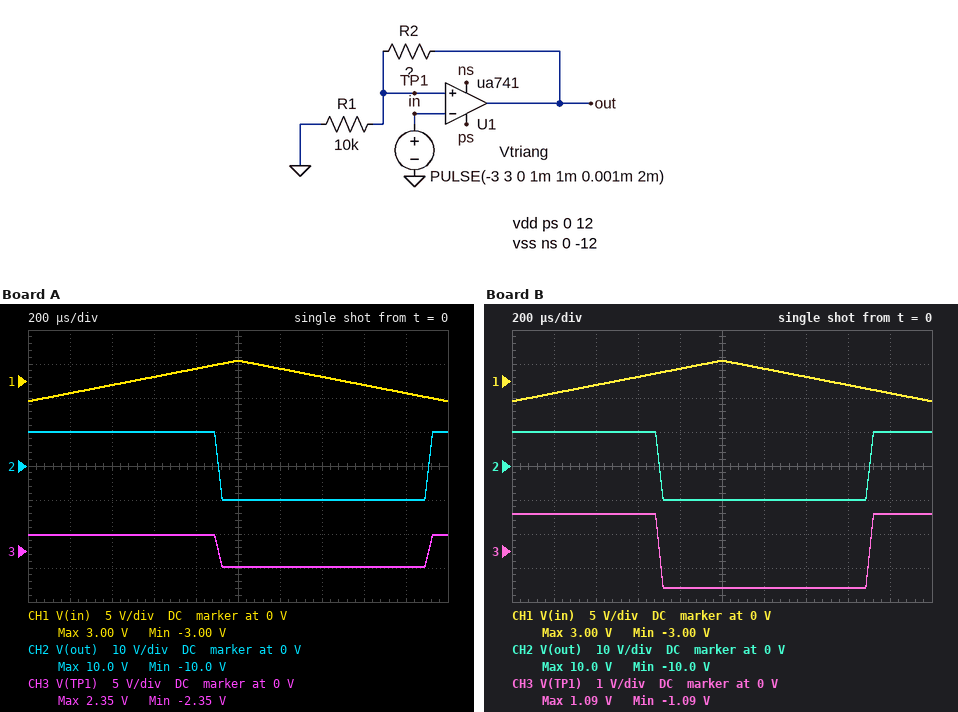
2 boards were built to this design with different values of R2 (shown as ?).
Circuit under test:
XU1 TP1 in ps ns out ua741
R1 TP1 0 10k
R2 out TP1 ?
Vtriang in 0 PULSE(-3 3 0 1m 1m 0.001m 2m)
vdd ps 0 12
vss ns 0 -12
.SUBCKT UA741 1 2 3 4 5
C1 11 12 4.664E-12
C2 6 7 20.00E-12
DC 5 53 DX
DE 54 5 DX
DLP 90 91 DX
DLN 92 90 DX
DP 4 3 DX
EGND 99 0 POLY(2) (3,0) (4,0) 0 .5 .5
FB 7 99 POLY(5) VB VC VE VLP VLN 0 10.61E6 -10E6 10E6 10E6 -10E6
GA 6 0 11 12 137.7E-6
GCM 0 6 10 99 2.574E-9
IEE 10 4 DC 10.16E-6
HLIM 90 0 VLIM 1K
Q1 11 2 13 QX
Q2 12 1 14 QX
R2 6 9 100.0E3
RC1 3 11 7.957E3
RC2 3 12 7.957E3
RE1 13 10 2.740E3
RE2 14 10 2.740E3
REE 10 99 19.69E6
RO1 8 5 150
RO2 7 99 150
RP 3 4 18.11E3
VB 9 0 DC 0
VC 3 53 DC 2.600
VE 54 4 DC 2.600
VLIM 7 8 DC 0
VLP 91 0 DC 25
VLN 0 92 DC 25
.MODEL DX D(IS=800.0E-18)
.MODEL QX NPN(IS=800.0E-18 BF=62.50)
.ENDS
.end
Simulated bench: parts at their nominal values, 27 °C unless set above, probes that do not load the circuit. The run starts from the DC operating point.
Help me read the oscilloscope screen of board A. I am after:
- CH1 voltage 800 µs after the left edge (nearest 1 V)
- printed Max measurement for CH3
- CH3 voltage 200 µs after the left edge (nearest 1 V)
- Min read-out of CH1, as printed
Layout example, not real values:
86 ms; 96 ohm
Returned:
2 V; 2.35 V; 2 V; -3.00 V
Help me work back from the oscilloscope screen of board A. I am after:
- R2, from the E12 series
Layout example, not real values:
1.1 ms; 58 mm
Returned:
33 kΩ
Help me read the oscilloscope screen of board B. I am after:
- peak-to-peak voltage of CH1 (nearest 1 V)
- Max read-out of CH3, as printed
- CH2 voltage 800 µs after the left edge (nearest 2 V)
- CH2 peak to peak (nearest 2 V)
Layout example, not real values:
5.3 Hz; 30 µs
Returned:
6 V; 1.09 V; -10 V; 20 V
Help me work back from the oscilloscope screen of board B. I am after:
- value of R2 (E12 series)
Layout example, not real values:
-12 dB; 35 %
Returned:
82 kΩ
